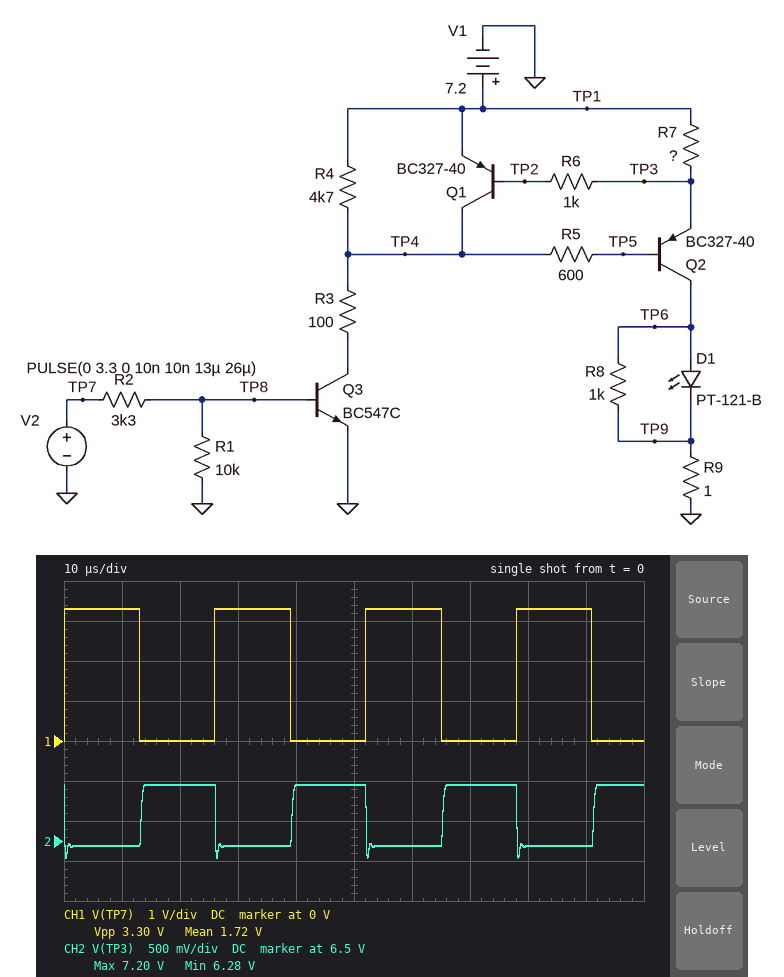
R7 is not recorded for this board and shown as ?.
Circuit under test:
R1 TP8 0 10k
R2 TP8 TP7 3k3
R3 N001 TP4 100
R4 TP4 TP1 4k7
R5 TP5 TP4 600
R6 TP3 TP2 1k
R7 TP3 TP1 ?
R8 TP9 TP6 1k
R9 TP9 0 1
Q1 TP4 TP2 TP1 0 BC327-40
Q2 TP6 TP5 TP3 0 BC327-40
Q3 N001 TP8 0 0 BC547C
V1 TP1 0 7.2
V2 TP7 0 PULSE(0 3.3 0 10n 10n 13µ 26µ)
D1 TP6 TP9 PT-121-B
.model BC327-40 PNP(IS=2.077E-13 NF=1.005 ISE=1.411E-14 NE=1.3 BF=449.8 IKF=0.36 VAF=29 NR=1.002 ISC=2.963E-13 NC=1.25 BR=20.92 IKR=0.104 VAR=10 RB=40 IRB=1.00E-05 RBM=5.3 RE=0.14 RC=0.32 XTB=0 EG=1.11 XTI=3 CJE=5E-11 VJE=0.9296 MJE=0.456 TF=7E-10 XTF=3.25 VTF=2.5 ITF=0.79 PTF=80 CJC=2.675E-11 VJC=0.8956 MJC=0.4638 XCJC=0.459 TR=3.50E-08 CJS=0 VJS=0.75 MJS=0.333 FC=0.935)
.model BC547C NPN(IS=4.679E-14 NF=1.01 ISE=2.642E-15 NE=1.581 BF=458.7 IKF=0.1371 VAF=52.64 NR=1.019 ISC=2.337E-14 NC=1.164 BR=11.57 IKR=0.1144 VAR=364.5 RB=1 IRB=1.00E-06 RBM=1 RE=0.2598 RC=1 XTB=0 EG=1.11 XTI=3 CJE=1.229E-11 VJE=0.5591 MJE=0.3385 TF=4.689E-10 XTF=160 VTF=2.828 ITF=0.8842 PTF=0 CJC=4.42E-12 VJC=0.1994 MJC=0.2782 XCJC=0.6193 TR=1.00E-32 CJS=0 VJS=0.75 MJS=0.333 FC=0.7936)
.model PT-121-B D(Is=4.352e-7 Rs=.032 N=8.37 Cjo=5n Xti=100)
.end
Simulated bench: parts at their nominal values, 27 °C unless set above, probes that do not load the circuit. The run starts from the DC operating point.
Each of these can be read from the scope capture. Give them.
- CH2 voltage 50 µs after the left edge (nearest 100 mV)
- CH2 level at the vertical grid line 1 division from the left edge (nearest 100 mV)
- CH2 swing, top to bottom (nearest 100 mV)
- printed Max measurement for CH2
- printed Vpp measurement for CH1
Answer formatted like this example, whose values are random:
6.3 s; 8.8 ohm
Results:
7.2 V; 6.4 V; 900 mV; 7.20 V; 3.30 V
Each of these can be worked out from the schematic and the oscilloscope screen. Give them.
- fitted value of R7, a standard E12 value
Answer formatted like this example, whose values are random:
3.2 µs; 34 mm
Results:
1.5 Ω
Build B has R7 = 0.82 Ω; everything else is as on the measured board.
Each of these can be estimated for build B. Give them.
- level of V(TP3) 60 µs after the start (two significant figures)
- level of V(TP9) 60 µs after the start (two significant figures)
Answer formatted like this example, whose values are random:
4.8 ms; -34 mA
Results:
6.5 V; 800 mV
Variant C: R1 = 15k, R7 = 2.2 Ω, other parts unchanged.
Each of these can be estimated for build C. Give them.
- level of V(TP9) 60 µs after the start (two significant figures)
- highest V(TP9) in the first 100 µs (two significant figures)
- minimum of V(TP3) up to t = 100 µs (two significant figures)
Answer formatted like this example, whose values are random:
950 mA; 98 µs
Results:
360 mV; 480 mV; 6.1 V
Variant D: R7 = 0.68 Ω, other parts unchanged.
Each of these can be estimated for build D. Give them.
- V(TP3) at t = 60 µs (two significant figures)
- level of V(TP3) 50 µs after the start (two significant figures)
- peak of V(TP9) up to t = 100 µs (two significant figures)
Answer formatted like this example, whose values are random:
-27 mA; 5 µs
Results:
6.6 V; 7.2 V; 890 mV
